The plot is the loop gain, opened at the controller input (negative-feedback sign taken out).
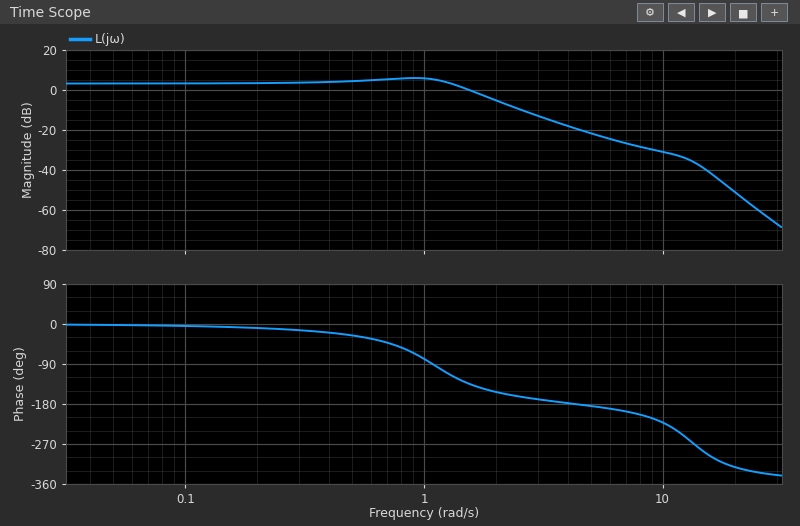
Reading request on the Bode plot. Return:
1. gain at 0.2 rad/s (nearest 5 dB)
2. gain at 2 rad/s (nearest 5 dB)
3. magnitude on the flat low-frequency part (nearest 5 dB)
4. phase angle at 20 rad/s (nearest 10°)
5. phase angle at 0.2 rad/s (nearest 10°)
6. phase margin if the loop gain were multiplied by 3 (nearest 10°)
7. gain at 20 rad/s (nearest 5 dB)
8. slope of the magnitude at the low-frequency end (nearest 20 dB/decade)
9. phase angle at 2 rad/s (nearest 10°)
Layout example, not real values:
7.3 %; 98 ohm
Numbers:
5 dB; -5 dB; 5 dB; -320°; -10°; 20°; -50 dB; 0 dB/decade; -150°
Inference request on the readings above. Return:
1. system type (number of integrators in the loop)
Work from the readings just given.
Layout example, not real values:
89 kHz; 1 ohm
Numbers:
0
